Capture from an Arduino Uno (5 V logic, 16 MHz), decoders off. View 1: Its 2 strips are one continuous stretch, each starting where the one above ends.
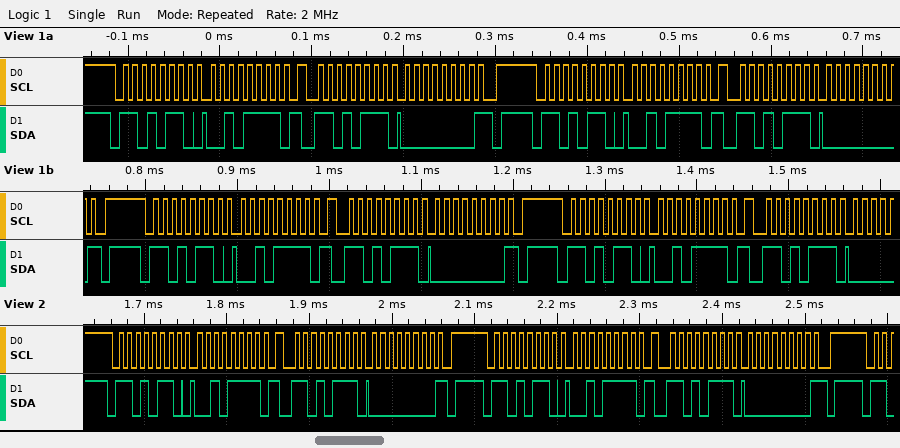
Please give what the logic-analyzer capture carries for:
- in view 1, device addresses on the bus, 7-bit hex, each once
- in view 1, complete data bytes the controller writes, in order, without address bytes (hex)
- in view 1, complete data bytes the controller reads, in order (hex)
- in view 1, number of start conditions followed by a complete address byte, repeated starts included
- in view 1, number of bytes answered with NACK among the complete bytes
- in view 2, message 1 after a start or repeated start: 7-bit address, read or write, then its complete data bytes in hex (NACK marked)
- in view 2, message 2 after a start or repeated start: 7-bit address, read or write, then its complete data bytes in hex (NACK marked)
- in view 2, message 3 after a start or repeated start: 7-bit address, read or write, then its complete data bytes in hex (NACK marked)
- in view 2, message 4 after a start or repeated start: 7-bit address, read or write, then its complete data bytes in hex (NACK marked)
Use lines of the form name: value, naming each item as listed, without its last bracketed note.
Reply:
in view 1, device addresses on the bus, 7-bit hex, each once: 0x6B
in view 1, complete data bytes the controller writes, in order, without address bytes: 2F 2F 2F 2F
in view 1, complete data bytes the controller reads, in order: 00 00 00
in view 1, number of start conditions followed by a complete address byte, repeated starts included: 8
in view 1, number of bytes answered with NACK among the complete bytes: 3
in view 2, message 1 after a start or repeated start: 7-bit address, read or write, then its complete data bytes in hex: 0x6B write: 2F
in view 2, message 2 after a start or repeated start: 7-bit address, read or write, then its complete data bytes in hex: 0x6B read: 00 NACK
in view 2, message 3 after a start or repeated start: 7-bit address, read or write, then its complete data bytes in hex: 0x6B write: 2F
in view 2, message 4 after a start or repeated start: 7-bit address, read or write, then its complete data bytes in hex: 0x6B read: 00 NACK
